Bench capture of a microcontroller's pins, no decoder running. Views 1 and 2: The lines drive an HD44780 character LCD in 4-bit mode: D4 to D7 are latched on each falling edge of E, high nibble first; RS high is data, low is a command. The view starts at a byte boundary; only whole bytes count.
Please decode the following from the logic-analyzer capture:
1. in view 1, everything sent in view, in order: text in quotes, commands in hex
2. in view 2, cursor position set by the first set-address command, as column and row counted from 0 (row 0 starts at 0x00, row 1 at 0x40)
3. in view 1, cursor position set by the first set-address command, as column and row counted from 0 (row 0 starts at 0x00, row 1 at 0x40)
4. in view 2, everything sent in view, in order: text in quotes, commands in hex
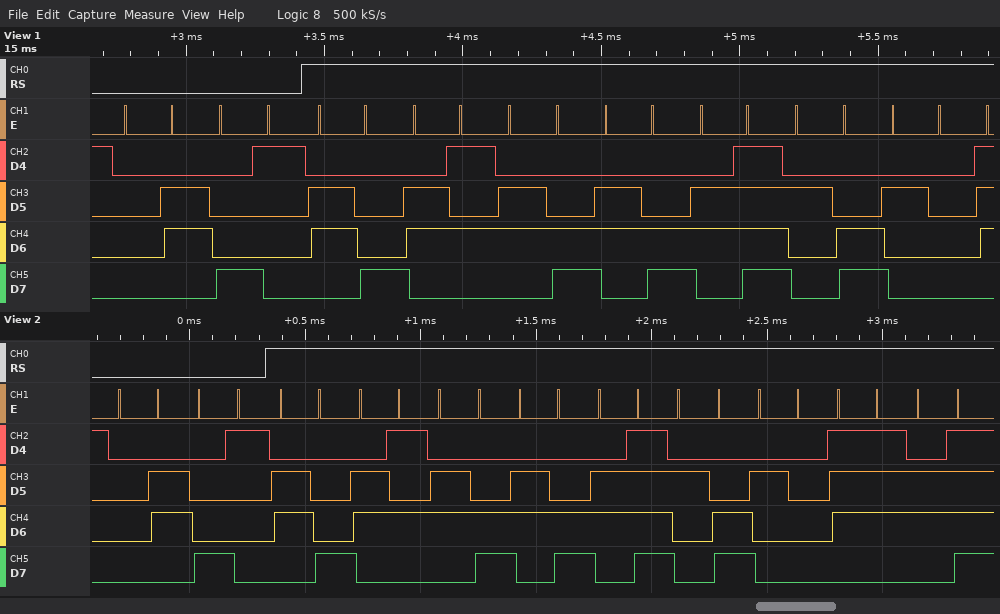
0x06 0x81 "hello, "
column 1, row 0
column 1, row 0
0x06 0x81 "hello, wo"
